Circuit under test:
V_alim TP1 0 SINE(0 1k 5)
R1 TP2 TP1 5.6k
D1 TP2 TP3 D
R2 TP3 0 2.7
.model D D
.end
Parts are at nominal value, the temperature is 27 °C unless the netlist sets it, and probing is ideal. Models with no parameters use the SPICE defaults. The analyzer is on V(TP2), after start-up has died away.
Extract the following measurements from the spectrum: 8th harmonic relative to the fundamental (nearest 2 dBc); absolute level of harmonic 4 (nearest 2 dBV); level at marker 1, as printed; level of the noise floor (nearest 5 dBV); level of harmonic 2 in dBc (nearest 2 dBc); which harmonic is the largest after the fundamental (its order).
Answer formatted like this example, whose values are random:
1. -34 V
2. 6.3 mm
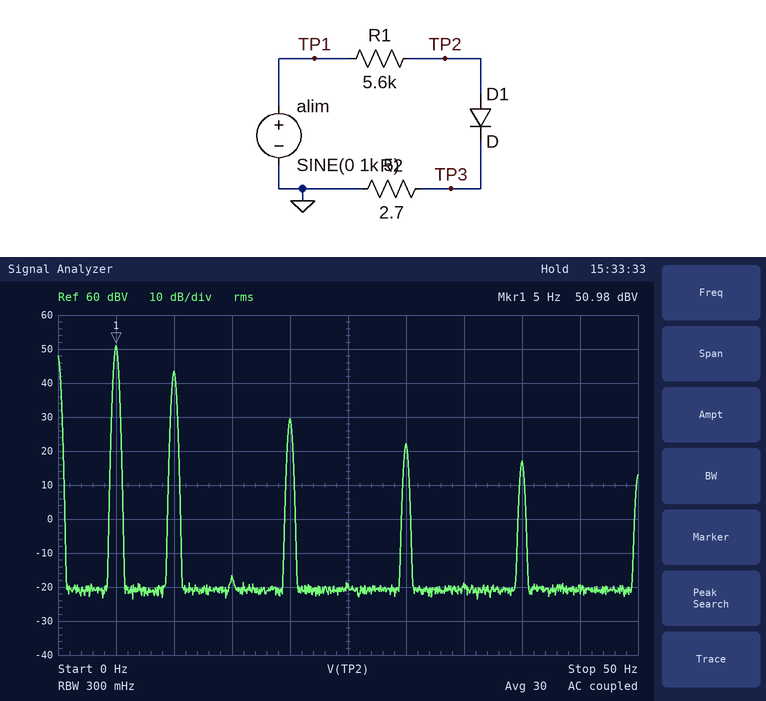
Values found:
1. -34 dBc
2. 30 dBV
3. 50.98 dBV
4. -20 dBV
5. -8 dBc
6. 2
